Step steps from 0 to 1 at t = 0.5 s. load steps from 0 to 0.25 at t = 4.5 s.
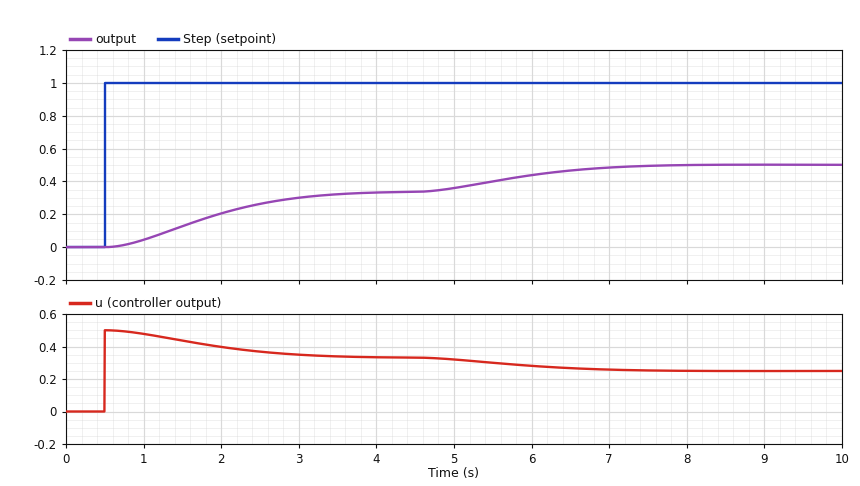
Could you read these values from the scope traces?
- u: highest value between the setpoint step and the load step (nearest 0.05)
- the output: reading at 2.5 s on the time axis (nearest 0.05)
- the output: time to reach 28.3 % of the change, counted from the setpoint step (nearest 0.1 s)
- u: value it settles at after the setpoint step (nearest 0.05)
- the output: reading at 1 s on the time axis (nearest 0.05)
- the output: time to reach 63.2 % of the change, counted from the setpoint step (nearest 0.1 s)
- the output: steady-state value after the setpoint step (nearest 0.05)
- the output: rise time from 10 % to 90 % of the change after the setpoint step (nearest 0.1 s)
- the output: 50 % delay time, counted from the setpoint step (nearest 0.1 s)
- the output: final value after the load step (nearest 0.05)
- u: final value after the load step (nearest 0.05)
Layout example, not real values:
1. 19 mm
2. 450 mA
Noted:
1. 0.50
2. 0.25
3. 0.8 s
4. 0.35
5. 0.05
6. 1.5 s
7. 0.35
8. 2.1 s
9. 1.2 s
10. 0.50
11. 0.25
